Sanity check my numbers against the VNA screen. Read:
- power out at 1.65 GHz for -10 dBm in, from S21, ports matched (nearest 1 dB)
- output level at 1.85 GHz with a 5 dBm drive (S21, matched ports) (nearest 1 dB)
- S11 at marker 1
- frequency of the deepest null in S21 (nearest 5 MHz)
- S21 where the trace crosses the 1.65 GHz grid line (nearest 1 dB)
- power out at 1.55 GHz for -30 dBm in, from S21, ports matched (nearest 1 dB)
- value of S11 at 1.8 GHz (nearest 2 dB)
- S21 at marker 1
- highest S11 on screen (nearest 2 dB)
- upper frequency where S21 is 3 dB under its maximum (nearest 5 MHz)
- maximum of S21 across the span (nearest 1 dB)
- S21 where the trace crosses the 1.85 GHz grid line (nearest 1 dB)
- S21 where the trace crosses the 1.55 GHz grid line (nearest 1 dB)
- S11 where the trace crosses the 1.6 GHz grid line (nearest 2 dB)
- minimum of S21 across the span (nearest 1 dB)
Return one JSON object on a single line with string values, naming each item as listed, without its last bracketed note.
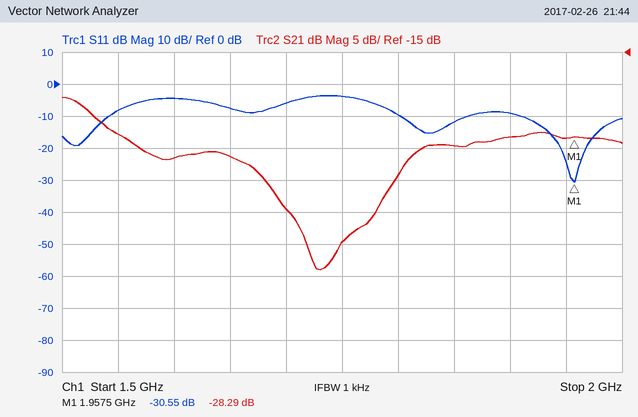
{"power out at 1.65 GHz for -10 dBm in, from S21, ports matched": "-41 dBm", "output level at 1.85 GHz with a 5 dBm drive (S21, matched ports)": "-25 dBm", "S11 at marker 1": "-30.55 dB", "frequency of the deepest null in S21": "1.730 GHz", "S21 where the trace crosses the 1.65 GHz grid line": "-31 dB", "power out at 1.55 GHz for -30 dBm in, from S21, ports matched": "-58 dBm", "value of S11 at 1.8 GHz": "-10 dB", "S21 at marker 1": "-28.29 dB", "highest S11 on screen": "-4 dB", "upper frequency where S21 is 3 dB under its maximum": "1.530 GHz", "maximum of S21 across the span": "-22 dB", "S21 where the trace crosses the 1.85 GHz grid line": "-30 dB", "S21 where the trace crosses the 1.55 GHz grid line": "-28 dB", "S11 where the trace crosses the 1.6 GHz grid line": "-4 dB", "minimum of S21 across the span": "-49 dB"}
